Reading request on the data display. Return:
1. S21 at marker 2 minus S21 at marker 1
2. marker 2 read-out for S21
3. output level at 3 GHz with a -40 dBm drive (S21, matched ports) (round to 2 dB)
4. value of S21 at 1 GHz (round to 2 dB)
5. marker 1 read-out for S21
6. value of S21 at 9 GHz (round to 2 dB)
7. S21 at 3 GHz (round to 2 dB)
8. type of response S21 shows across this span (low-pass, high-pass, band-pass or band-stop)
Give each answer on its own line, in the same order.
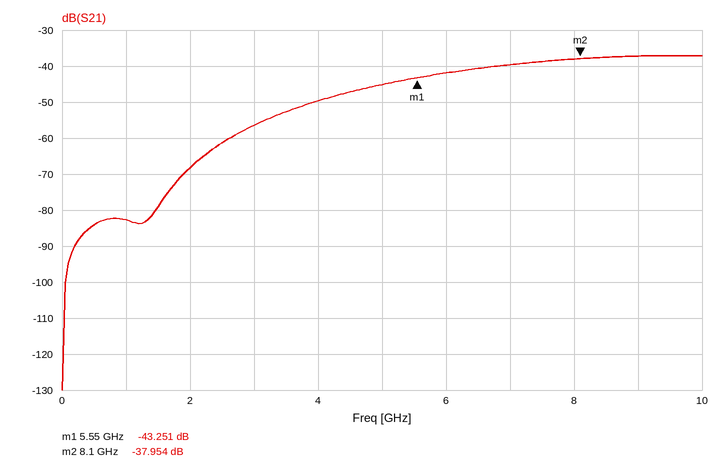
5.297 dB
-37.954 dB
-96 dBm
-82 dB
-43.251 dB
-38 dB
-56 dB
high-pass
